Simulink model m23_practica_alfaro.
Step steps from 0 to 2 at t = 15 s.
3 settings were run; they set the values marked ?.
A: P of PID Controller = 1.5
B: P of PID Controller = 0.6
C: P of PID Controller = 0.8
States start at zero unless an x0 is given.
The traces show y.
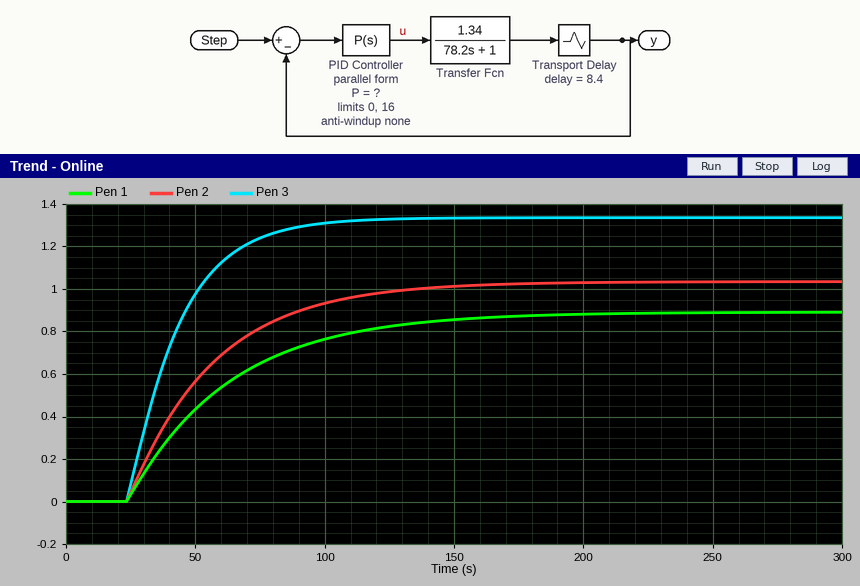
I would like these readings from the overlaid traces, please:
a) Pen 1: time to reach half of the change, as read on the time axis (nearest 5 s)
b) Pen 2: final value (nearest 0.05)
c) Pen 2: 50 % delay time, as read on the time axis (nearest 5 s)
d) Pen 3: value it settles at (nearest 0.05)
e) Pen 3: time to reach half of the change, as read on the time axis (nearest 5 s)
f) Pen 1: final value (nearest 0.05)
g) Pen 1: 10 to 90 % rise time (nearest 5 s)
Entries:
50 s
1.05
45 s
1.35
40 s
0.90
85 s
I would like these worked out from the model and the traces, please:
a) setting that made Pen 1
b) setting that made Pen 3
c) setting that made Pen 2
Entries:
B
A
C
